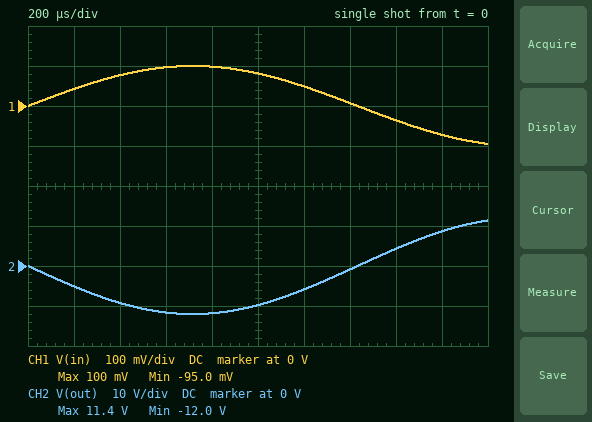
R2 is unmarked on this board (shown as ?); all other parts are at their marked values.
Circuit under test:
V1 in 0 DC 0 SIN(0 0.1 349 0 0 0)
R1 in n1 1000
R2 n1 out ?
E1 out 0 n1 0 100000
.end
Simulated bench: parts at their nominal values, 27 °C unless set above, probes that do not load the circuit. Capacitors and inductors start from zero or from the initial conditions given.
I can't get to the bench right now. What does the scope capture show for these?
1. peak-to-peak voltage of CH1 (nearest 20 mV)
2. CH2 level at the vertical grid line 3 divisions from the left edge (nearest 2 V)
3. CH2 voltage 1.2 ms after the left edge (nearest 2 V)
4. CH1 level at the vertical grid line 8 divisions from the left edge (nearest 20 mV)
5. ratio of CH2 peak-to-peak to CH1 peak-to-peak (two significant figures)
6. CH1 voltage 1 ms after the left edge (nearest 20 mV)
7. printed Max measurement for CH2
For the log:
200 mV
-12 V
-6 V
-40 mV
120
80 mV
11.4 V
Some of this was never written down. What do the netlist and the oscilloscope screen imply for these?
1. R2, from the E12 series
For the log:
120 kΩ
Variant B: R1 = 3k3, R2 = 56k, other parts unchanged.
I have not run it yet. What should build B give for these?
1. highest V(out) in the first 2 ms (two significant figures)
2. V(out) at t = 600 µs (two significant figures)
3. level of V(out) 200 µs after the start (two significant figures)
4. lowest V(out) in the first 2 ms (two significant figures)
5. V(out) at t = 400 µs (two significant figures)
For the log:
1.6 V
-1.6 V
-720 mV
-1.7 V
-1.3 V
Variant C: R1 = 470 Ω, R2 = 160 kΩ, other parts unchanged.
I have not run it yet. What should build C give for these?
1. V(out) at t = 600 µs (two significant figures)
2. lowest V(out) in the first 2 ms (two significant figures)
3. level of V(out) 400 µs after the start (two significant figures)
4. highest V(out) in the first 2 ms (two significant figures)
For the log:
-33 V
-34 V
-26 V
32 V
